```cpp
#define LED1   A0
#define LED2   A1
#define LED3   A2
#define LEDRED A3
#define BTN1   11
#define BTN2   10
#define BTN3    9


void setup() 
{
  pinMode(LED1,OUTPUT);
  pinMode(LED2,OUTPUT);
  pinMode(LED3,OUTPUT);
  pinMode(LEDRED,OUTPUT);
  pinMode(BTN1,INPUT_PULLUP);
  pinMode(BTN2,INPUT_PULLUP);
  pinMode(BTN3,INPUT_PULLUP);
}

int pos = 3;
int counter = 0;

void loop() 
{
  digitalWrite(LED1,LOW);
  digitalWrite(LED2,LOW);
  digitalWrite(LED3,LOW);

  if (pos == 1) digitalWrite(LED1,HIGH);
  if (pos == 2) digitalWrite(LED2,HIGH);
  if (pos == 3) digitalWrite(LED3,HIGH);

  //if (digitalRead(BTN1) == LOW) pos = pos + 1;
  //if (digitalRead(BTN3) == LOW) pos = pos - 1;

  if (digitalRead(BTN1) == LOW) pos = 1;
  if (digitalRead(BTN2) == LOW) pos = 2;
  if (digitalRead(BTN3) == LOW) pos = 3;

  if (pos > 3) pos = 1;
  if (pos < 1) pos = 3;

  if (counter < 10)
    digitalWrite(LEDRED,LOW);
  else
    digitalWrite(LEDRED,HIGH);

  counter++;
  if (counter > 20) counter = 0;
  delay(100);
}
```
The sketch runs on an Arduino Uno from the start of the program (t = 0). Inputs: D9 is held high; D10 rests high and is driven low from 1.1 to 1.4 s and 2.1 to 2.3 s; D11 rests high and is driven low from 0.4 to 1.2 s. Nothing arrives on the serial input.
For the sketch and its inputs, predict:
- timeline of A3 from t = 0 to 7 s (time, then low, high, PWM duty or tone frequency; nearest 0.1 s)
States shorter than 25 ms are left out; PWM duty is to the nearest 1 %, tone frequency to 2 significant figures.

0 s low; 1 s high; 2.1 s low; 3.1 s high; 4.2 s low; 5.2 s high; 6.3 s low
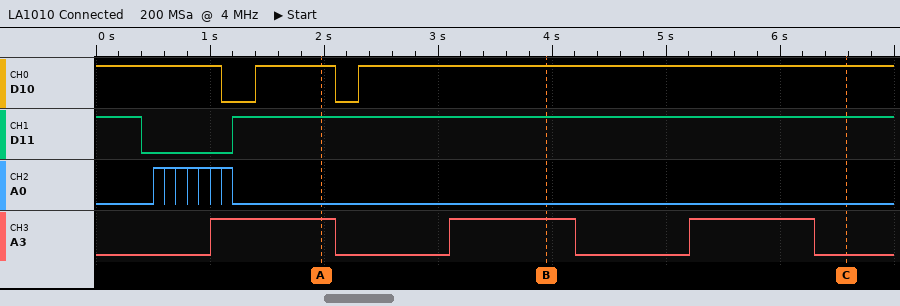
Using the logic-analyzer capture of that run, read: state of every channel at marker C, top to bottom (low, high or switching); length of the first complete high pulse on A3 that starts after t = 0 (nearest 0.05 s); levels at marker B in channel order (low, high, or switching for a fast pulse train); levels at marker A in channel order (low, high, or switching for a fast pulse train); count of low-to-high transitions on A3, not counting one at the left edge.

D10 high, D11 high, A0 low, A3 low
1.10 s
D10 high, D11 high, A0 low, A3 high
D10 high, D11 high, A0 low, A3 high
3
